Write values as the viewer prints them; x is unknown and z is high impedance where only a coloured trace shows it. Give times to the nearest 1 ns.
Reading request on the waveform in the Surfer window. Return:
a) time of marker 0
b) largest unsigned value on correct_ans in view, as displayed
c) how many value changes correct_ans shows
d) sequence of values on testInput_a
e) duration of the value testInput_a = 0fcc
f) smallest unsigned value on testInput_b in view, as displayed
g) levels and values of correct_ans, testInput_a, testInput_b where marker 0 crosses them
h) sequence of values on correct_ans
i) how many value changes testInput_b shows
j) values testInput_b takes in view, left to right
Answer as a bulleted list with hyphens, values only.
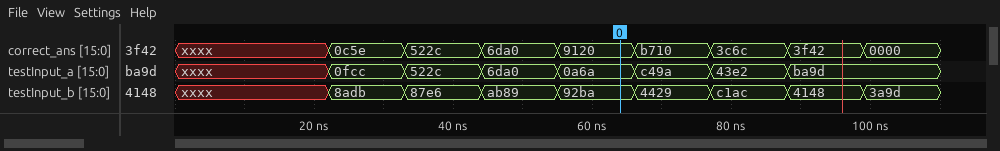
- 64 ns
- b710
- 8
- xxxx, 0fcc, 522c, 6da0, 0a6a, c49a, 43e2, ba9d
- 11 ns
- 3a9d
- correct_ans=9120, testInput_a=0a6a, testInput_b=92ba
- xxxx, 0c5e, 522c, 6da0, 9120, b710, 3c6c, 3f42, 0000
- 8
- xxxx, 8adb, 87e6, ab89, 92ba, 4429, c1ac, 4148, 3a9d
